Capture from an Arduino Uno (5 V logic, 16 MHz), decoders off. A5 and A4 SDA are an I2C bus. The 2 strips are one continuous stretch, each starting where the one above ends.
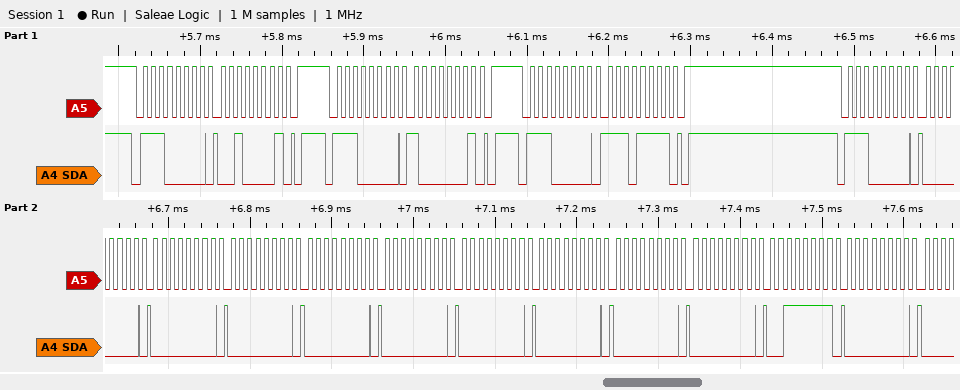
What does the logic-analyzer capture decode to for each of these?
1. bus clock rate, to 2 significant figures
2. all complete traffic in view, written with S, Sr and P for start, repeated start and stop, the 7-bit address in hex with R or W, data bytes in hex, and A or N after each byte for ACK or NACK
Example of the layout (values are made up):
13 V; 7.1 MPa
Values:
100 kHz; S 70W A 21 A P S 70W A 81 A P S 70W A EF A P S 70W A 00 A 00 A 00 A 00 A 00 A 00 A 00 A 00 A 00 A 3F A 00 A
